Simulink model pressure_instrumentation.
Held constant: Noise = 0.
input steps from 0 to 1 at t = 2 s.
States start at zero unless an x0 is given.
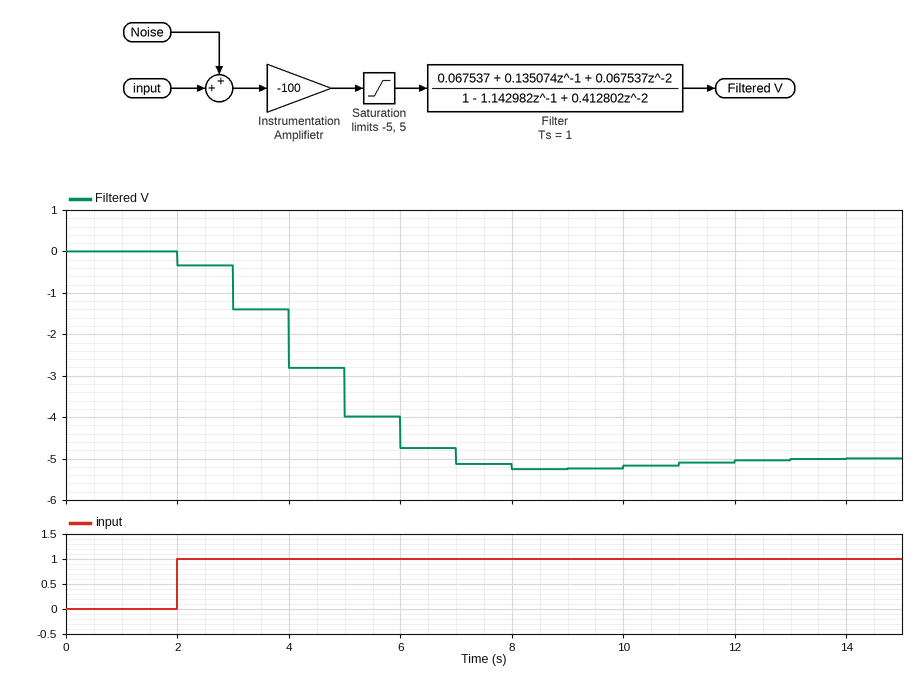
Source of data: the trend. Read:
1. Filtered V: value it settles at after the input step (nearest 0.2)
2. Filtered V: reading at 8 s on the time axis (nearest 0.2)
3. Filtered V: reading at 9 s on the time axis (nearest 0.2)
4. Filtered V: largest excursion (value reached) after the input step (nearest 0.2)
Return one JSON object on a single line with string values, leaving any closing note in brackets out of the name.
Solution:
{"Filtered V: value it settles at after the input step": "-5.0", "Filtered V: reading at 8 s on the time axis": "-5.2", "Filtered V: reading at 9 s on the time axis": "-5.2", "Filtered V: largest excursion (value reached) after the input step": "-5.2"}
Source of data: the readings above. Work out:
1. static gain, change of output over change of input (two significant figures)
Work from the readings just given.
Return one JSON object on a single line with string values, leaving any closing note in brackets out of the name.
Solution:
{"static gain, change of output over change of input": "-5.0"}
